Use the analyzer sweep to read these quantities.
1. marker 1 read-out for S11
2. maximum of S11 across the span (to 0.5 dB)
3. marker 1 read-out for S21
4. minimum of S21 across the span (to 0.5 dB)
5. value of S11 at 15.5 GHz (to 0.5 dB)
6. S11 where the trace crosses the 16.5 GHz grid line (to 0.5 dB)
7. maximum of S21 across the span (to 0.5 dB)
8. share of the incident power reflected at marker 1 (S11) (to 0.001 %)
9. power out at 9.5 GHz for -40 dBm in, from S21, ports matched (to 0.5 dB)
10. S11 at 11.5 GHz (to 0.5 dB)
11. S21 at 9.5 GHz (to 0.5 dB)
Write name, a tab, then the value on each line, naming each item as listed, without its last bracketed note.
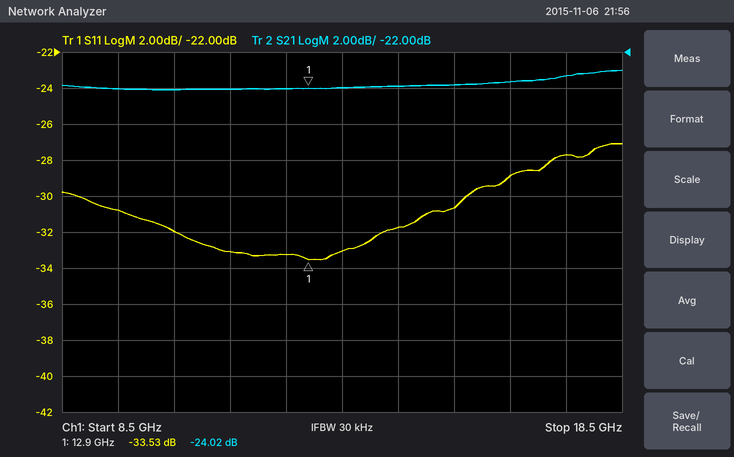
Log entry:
marker 1 read-out for S11	-33.53 dB
maximum of S11 across the span	-27.0 dB
marker 1 read-out for S21	-24.02 dB
minimum of S21 across the span	-24.0 dB
value of S11 at 15.5 GHz	-30.5 dB
S11 where the trace crosses the 16.5 GHz grid line	-29.0 dB
maximum of S21 across the span	-23.0 dB
share of the incident power reflected at marker 1 (S11)	0.044 %
power out at 9.5 GHz for -40 dBm in, from S21, ports matched	-64.0 dBm
S11 at 11.5 GHz	-33.0 dB
S21 at 9.5 GHz	-24.0 dB
